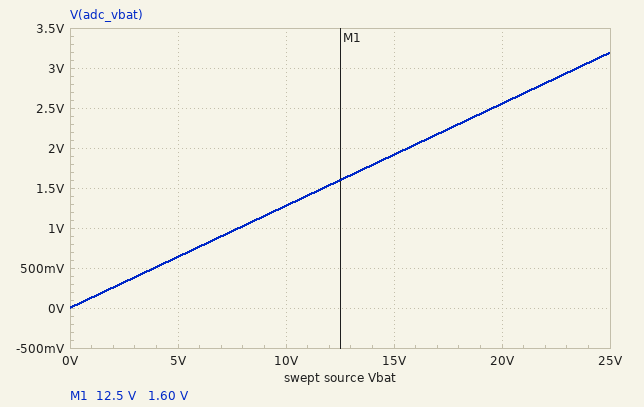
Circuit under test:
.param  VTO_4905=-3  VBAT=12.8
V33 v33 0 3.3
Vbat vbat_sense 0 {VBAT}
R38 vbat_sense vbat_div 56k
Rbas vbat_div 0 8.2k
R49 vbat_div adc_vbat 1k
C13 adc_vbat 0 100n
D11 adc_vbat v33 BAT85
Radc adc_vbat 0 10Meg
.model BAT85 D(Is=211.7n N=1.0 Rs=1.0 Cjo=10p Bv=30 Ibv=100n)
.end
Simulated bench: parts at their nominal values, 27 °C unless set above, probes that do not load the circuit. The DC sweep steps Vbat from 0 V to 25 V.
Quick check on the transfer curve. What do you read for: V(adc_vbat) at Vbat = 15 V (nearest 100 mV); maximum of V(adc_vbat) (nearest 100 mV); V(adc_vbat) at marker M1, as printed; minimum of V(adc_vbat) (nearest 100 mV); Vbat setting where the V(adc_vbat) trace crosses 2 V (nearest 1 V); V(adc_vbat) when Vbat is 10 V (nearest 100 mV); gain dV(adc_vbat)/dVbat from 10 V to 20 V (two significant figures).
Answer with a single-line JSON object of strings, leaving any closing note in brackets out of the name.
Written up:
{"V(adc_vbat) at Vbat = 15 V": "1.9 V", "maximum of V(adc_vbat)": "3.2 V", "V(adc_vbat) at marker M1, as printed": "1.60 V", "minimum of V(adc_vbat)": "0 V", "Vbat setting where the V(adc_vbat) trace crosses 2 V": "16 V", "V(adc_vbat) when Vbat is 10 V": "1.3 V", "gain dV(adc_vbat)/dVbat from 10 V to 20 V": "0.13 V/V"}
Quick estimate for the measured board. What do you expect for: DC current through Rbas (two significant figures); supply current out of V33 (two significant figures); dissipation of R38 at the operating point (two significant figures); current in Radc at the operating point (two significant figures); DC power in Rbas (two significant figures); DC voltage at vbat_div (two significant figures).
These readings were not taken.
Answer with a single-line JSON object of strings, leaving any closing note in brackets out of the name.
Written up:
{"DC current through Rbas": "200 µA", "supply current out of V33": "210 nA", "dissipation of R38 at the operating point": "2.2 mW", "current in Radc at the operating point": "160 nA", "DC power in Rbas": "330 µW", "DC voltage at vbat_div": "1.6 V"}
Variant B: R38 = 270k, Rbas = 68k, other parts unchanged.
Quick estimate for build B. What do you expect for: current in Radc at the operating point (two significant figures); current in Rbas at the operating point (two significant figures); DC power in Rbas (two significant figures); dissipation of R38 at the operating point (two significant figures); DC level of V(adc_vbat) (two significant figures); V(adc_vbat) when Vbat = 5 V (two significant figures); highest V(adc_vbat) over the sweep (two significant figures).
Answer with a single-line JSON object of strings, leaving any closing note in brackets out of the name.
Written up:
{"current in Radc at the operating point": "260 nA", "current in Rbas at the operating point": "38 µA", "DC power in Rbas": "97 µW", "dissipation of R38 at the operating point": "390 µW", "DC level of V(adc_vbat)": "2.6 V", "V(adc_vbat) when Vbat = 5 V": "1.0 V", "highest V(adc_vbat) over the sweep": "3.4 V"}
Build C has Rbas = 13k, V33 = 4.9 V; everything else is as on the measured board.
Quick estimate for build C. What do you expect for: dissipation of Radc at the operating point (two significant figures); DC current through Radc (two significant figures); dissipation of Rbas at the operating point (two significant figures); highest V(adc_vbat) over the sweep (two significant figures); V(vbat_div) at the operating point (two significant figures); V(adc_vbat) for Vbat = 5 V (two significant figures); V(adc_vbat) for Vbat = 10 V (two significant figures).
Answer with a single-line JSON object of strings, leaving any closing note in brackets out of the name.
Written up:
{"dissipation of Radc at the operating point": "580 nW", "DC current through Radc": "240 nA", "dissipation of Rbas at the operating point": "450 µW", "highest V(adc_vbat) over the sweep": "4.7 V", "V(vbat_div) at the operating point": "2.4 V", "V(adc_vbat) for Vbat = 5 V": "940 mV", "V(adc_vbat) for Vbat = 10 V": "1.9 V"}
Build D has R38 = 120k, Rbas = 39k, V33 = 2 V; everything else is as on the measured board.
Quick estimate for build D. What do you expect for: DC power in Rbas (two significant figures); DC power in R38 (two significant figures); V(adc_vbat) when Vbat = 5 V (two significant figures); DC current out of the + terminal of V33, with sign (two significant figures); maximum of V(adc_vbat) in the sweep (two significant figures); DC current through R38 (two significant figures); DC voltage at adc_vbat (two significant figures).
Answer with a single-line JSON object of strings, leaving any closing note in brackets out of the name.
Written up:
{"DC power in Rbas": "120 µW", "DC power in R38": "940 µW", "V(adc_vbat) when Vbat = 5 V": "1.2 V", "DC current out of the + terminal of V33, with sign": "-33 µA", "maximum of V(adc_vbat) in the sweep": "2.2 V", "DC current through R38": "89 µA", "DC voltage at adc_vbat": "2.1 V"}
